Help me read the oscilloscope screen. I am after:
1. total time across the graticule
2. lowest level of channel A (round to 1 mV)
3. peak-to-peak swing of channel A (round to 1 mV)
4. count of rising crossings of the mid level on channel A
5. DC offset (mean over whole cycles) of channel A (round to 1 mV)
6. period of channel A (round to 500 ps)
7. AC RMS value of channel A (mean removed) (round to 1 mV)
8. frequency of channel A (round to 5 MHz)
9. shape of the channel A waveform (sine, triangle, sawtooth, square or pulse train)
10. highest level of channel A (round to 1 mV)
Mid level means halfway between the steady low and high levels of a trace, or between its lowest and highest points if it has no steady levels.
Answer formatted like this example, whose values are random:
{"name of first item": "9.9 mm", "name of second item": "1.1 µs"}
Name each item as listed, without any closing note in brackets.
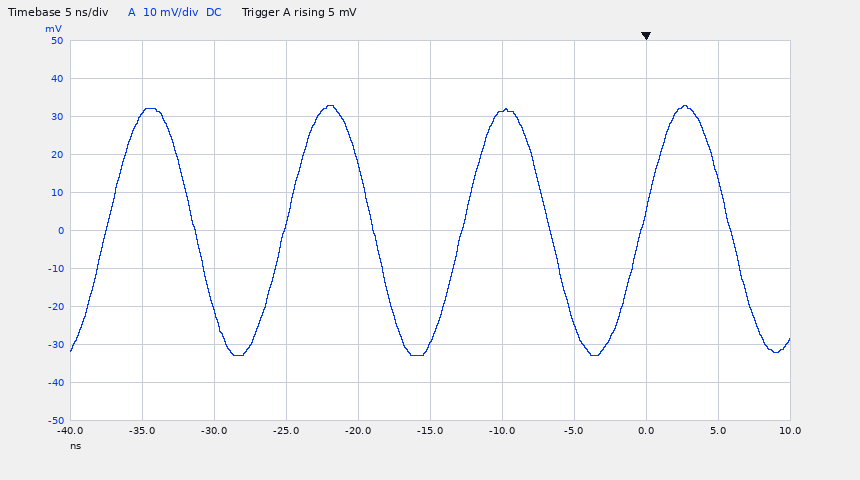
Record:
{"total time across the graticule": "50 ns", "lowest level of channel A": "-33 mV", "peak-to-peak swing of channel A": "66 mV", "count of rising crossings of the mid level on channel A": "4", "DC offset (mean over whole cycles) of channel A": "0 mV", "period of channel A": "12.5 ns", "AC RMS value of channel A (mean removed)": "23 mV", "frequency of channel A": "80 MHz", "shape of the channel A waveform": "sine", "highest level of channel A": "33 mV"}
